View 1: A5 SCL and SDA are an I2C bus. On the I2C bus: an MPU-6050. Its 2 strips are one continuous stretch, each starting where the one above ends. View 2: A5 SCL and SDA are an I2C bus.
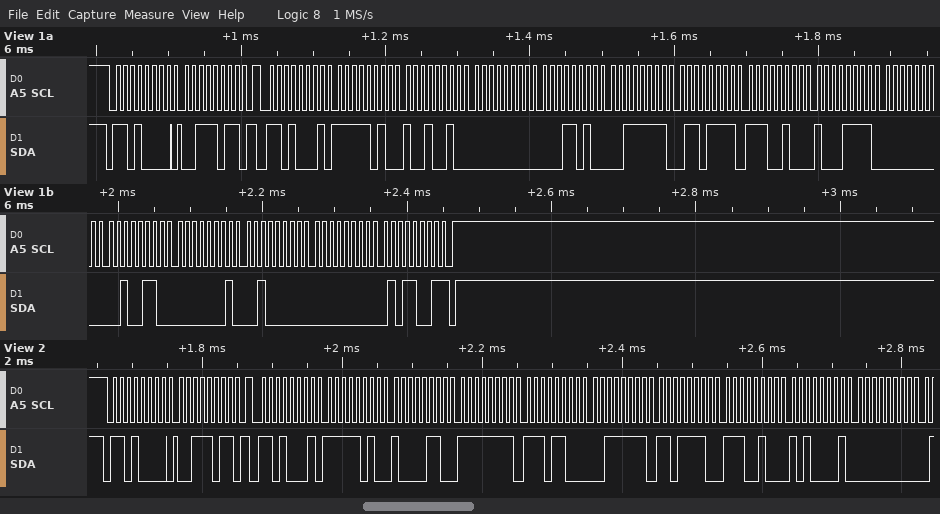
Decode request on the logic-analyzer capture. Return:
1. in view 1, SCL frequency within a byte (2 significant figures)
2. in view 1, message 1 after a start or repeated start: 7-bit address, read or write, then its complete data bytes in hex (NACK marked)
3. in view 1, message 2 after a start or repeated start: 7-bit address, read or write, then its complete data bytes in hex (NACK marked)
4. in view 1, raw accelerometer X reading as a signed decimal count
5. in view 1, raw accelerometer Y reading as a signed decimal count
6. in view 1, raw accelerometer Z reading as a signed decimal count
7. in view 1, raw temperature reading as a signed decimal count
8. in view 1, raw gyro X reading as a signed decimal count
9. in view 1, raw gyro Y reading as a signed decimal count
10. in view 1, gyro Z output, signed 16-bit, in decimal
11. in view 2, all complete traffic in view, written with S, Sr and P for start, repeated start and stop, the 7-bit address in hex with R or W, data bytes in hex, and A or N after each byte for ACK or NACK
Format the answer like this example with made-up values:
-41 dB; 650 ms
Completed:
100 kHz; 0x68 write: 3B; 0x68 read: FA 92 00 1A 3F 6F E4 8F 00 26 01 20 00 59 NACK; -1390; 26; 16239; -7025; 38; 288; 89; S 68W A 3B A Sr 68R A FA A 86 A FF A EC A 3F A DE A E4 A A1 A 00 A
